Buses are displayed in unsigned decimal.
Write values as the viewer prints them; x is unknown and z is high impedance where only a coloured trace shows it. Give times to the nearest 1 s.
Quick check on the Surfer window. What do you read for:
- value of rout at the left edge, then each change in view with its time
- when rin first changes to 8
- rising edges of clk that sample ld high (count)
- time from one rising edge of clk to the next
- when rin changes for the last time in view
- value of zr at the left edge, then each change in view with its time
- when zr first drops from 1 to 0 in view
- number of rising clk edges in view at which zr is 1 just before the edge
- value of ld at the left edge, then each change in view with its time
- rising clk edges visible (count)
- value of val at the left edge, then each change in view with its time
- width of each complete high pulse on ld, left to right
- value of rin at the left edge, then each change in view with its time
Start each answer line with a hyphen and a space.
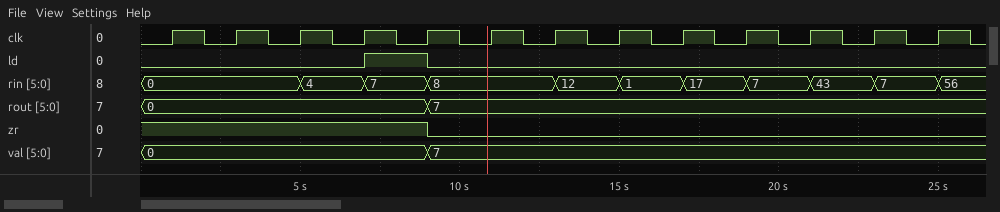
- 0, 7 at 9 s
- 9 s
- 1
- 2 s
- 25 s
- 1, 0 at 9 s
- 9 s
- 5
- 0, 1 at 7 s, 0 at 9 s
- 13
- 0, 7 at 9 s
- 2 s
- 0, 4 at 5 s, 7 at 7 s, 8 at 9 s, 12 at 13 s, 1 at 15 s, 17 at 17 s, 7 at 19 s, 43 at 21 s, 7 at 23 s, 56 at 25 s
